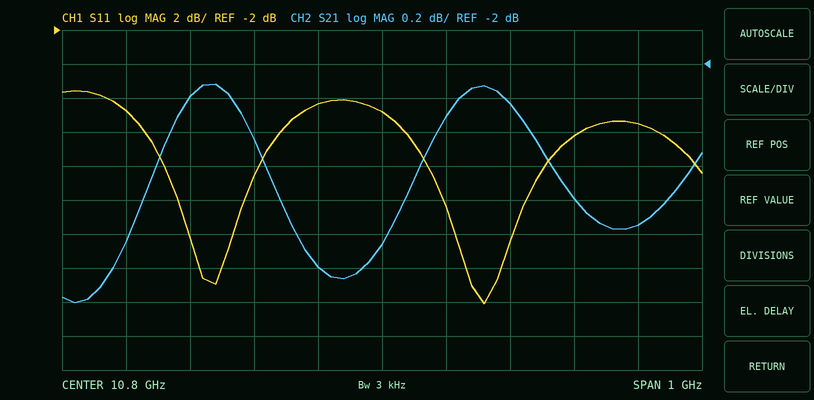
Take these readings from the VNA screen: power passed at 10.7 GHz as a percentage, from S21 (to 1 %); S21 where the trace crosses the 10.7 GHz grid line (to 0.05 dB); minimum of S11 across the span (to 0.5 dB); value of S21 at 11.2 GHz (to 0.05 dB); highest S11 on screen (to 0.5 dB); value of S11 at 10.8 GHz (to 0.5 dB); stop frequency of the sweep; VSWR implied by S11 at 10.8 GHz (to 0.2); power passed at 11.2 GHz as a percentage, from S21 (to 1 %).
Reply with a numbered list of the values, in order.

1. 48 %
2. -3.20 dB
3. -18.0 dB
4. -2.95 dB
5. -5.5 dB
6. -7.0 dB
7. 11.3 GHz
8. 2.6
9. 51 %
